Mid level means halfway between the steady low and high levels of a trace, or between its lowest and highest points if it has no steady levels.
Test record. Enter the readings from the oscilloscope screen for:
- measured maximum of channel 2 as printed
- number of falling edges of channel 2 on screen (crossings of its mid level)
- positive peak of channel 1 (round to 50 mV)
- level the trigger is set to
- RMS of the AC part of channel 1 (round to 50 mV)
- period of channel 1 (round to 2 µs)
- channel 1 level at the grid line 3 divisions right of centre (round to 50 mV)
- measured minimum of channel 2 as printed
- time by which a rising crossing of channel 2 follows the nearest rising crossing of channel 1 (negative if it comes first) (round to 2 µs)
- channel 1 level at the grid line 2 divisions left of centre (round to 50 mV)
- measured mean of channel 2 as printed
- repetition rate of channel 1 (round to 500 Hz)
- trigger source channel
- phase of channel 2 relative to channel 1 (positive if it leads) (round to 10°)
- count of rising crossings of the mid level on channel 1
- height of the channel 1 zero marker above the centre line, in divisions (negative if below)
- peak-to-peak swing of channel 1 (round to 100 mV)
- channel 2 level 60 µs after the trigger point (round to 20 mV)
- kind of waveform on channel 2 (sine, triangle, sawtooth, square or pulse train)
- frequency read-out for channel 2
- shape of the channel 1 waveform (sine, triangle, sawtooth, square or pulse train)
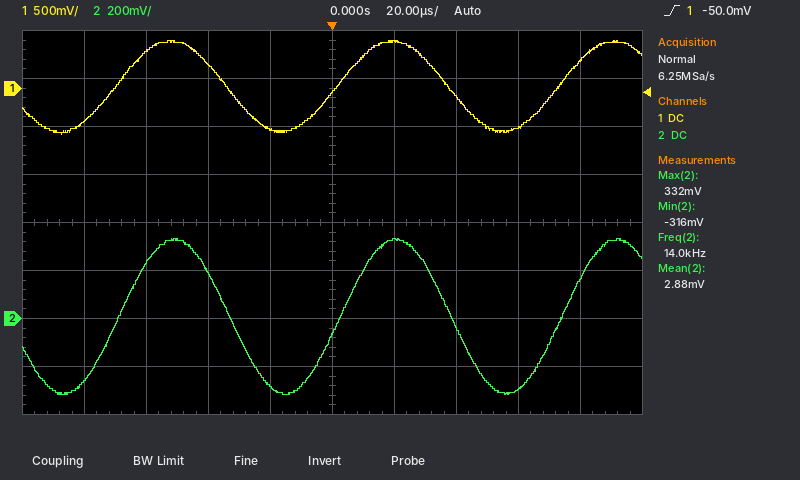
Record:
332 mV
2
500 mV
-50.0 mV
350 mV
72 µs
-400 mV
-316 mV
+2 µs
250 mV
2.88 mV
14.0 kHz
channel 1
-10°
3
+2.8 div
1.00 V
-300 mV
sine
14.0 kHz
sine
